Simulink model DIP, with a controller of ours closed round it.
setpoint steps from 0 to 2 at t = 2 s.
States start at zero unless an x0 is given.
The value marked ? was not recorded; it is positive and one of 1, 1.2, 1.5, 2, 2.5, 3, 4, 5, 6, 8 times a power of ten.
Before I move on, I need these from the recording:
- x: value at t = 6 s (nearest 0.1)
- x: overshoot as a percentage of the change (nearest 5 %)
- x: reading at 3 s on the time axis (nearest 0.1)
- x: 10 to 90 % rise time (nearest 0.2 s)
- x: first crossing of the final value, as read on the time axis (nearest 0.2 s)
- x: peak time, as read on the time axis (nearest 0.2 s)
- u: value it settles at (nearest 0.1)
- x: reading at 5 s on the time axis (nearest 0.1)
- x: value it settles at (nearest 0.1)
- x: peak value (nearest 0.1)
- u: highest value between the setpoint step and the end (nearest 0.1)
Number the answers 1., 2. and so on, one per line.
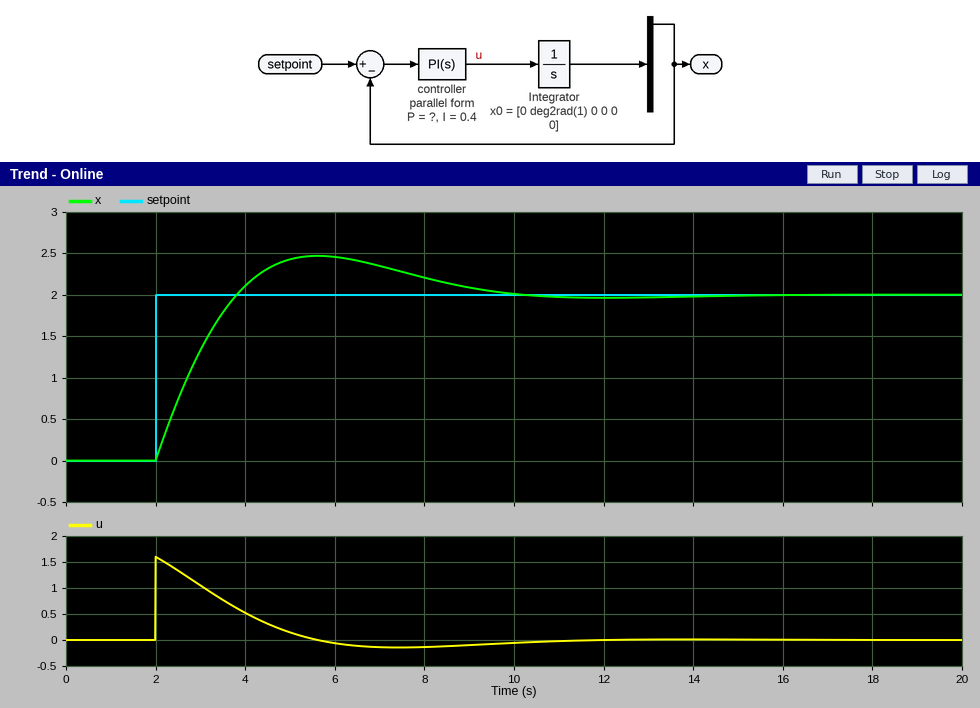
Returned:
1. 2.5
2. 25 %
3. 1.3
4. 1.4 s
5. 3.8 s
6. 5.6 s
7. 0.0
8. 2.4
9. 2.0
10. 2.5
11. 1.6
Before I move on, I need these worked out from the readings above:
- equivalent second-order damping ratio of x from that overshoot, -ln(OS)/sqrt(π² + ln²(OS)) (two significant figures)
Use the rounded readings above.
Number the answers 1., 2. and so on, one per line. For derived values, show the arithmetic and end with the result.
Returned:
1. ln(0.25) = -1.386; 1.386 / sqrt(9.870 + 1.922) = 0.40
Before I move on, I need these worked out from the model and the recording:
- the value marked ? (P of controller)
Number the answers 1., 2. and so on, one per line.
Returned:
1. 0.8
